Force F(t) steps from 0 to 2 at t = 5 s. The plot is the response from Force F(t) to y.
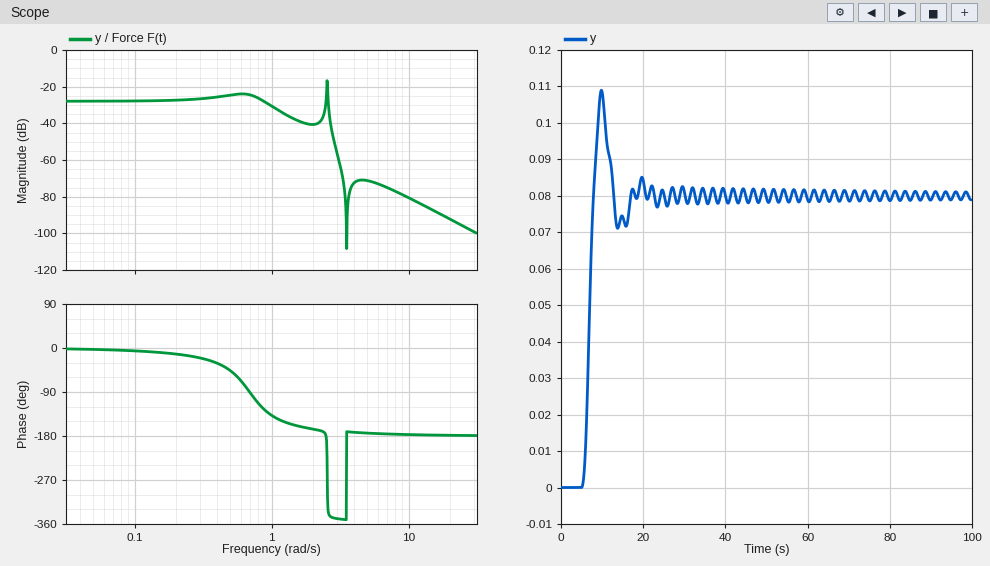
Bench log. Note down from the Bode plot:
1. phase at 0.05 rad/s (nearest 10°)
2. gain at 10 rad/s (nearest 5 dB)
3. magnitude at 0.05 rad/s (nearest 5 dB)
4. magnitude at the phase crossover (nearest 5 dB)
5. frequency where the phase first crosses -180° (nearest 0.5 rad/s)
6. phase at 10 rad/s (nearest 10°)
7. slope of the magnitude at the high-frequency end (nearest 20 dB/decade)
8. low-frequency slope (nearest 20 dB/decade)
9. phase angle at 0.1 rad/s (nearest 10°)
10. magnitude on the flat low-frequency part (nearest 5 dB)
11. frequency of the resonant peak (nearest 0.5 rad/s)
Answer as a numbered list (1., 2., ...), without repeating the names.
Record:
1. 0°
2. -80 dB
3. -30 dB
4. -30 dB
5. 2.5 rad/s
6. -180°
7. -40 dB/decade
8. 0 dB/decade
9. -10°
10. -30 dB
11. 2.5 rad/s
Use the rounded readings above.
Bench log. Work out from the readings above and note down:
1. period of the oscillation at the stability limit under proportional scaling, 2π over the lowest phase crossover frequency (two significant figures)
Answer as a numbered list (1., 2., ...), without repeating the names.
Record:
1. 2.5 s
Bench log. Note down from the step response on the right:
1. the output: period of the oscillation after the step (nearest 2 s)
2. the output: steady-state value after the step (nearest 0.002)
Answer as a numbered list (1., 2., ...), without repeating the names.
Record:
1. 10 s
2. 0.080
